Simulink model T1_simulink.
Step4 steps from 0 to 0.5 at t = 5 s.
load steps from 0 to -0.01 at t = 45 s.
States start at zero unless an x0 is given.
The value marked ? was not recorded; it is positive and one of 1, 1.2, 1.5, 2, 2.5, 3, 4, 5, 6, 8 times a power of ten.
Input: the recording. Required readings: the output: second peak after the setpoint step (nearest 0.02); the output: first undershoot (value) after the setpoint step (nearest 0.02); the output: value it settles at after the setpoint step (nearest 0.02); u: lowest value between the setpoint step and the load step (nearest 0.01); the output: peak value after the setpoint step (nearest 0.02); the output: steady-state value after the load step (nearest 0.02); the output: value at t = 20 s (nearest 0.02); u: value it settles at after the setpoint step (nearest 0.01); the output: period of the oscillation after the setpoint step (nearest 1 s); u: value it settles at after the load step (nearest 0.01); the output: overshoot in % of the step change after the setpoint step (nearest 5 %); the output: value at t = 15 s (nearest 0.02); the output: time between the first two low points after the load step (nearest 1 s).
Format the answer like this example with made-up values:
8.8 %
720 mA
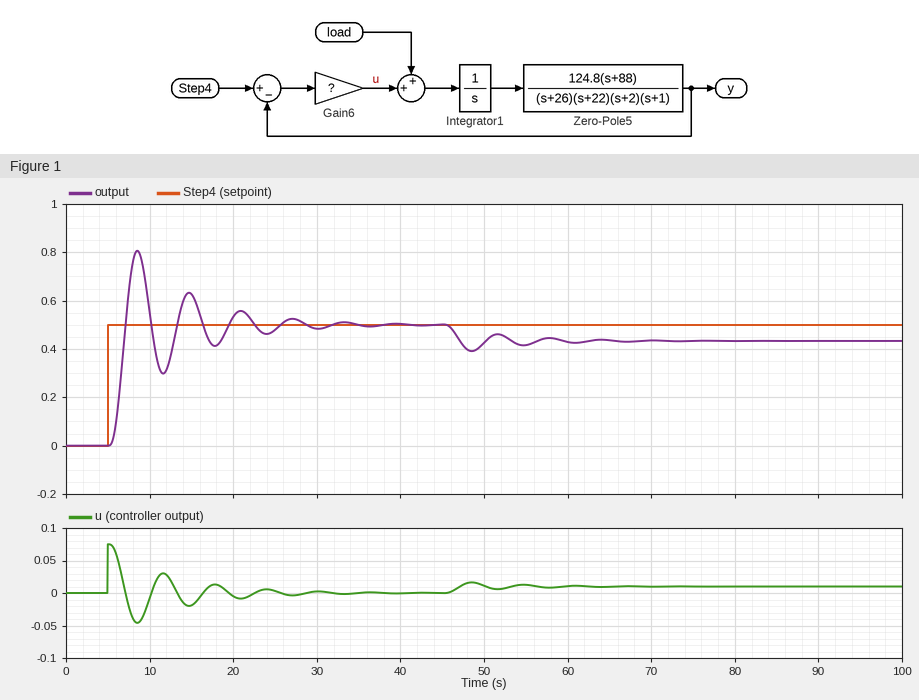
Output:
0.64
0.30
0.50
-0.05
0.80
0.44
0.54
0.00
6 s
0.01
60 %
0.62
6 s
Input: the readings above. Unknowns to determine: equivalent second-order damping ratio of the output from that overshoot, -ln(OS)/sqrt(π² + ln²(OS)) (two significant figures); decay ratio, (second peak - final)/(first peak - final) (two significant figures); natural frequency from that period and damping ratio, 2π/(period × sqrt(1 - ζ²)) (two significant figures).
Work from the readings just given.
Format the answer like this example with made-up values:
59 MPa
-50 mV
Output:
0.16
0.47
1.1 rad/s
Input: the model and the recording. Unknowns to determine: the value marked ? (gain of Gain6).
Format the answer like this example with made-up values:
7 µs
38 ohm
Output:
0.15
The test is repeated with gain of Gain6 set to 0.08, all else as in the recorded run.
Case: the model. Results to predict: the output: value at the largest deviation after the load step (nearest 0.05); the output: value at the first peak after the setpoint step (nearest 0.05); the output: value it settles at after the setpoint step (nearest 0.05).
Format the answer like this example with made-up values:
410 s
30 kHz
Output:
0.35
0.65
0.50
